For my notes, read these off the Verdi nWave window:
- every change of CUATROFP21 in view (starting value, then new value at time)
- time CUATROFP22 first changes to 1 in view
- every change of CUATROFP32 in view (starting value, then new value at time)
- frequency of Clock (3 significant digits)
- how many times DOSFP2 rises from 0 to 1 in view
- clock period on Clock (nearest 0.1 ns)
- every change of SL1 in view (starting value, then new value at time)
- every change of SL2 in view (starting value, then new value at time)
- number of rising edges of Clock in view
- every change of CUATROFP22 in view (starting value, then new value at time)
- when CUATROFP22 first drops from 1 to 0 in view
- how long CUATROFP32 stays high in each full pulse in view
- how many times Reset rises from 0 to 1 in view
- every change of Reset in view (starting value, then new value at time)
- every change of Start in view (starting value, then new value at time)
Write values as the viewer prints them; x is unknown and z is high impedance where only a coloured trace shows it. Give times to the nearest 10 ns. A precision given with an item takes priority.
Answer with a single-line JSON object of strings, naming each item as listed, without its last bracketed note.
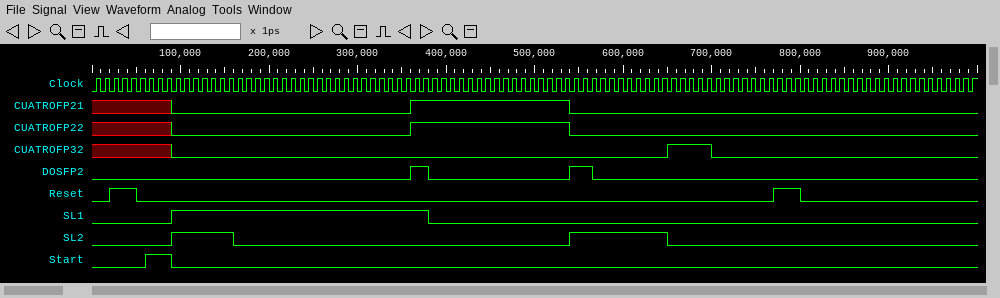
{"every change of CUATROFP21 in view": "x, 0 at 90 ns, 1 at 360 ns, 0 at 540 ns", "time CUATROFP22 first changes to 1 in view": "360 ns", "every change of CUATROFP32 in view": "x, 0 at 90 ns, 1 at 650 ns, 0 at 700 ns", "frequency of Clock": "100 MHz", "how many times DOSFP2 rises from 0 to 1 in view": "2", "clock period on Clock": "10 ns", "every change of SL1 in view": "0, 1 at 90 ns, 0 at 380 ns", "every change of SL2 in view": "0, 1 at 90 ns, 0 at 160 ns, 1 at 540 ns, 0 at 650 ns", "number of rising edges of Clock in view": "100", "every change of CUATROFP22 in view": "x, 0 at 90 ns, 1 at 360 ns, 0 at 540 ns", "when CUATROFP22 first drops from 1 to 0 in view": "540 ns", "how long CUATROFP32 stays high in each full pulse in view": "50 ns", "how many times Reset rises from 0 to 1 in view": "2", "every change of Reset in view": "0, 1 at 20 ns, 0 at 50 ns, 1 at 770 ns, 0 at 800 ns", "every change of Start in view": "0, 1 at 60 ns, 0 at 90 ns"}
